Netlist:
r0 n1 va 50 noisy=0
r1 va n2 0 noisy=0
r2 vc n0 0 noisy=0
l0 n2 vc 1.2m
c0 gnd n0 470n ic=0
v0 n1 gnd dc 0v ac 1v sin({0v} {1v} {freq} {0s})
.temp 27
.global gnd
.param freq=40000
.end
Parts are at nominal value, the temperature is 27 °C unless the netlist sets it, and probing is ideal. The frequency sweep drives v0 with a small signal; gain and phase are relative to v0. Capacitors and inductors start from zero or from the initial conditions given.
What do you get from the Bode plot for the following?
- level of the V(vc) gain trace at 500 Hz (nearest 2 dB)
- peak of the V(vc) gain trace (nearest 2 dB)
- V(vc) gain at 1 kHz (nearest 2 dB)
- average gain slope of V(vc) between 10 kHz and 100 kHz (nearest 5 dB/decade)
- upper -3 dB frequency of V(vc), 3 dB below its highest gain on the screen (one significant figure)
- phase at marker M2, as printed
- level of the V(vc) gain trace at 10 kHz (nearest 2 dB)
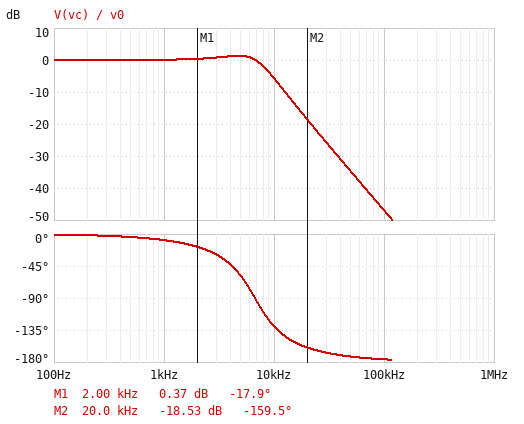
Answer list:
0 dB
2 dB
0 dB
-40 dB/decade
8 kHz
-159.5 deg
-6 dB
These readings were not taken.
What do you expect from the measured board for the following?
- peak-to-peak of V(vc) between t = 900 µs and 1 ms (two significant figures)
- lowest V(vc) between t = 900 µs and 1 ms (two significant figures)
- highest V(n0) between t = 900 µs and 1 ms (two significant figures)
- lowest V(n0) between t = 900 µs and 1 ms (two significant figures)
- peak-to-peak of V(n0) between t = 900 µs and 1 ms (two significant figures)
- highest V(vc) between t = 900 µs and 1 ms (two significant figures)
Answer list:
57 mV
-28 mV
28 mV
-28 mV
57 mV
28 mV
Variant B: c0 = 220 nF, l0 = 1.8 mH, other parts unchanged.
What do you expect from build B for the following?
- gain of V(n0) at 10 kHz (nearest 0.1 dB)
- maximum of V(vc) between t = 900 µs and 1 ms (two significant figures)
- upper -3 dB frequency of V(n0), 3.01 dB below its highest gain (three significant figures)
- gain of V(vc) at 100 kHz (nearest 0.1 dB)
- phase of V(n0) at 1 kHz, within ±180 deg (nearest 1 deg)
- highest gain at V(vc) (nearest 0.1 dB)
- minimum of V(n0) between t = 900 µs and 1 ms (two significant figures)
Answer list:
1.0 dB
41 mV
9.39 kHz
-43.8 dB
-4 deg
5.5 dB
-41 mV
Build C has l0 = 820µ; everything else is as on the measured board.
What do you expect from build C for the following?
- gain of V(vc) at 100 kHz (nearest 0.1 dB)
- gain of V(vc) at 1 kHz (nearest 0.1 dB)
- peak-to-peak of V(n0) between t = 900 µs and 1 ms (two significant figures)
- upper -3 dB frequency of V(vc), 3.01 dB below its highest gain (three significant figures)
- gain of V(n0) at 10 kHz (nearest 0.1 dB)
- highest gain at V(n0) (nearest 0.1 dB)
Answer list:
-43.6 dB
0 dB
83 mV
9.04 kHz
-3.9 dB
0.4 dB
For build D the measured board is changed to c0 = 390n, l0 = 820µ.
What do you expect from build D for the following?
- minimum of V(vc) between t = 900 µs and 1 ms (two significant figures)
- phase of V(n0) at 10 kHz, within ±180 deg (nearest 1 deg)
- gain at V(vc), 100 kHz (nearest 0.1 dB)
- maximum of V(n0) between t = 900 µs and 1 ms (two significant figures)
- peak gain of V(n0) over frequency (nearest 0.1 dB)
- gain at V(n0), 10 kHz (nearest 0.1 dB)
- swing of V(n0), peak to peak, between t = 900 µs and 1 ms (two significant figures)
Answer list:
-50 mV
-102 deg
-42.0 dB
50 mV
0.8 dB
-2.0 dB
100 mV
